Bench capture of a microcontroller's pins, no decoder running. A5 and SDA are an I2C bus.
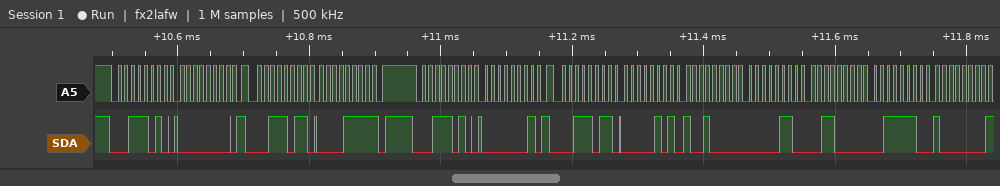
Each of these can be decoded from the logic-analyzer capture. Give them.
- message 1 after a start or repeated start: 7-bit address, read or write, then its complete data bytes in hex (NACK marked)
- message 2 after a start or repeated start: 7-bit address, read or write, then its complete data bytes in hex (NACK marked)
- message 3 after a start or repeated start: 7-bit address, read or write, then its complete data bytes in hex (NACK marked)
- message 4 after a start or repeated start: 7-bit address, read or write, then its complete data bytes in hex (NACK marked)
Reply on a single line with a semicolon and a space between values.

0x1D write: 00; 0x1D read: 0F NACK; 0x1D write: 01; 0x1D read: 05 90 06 30 3E 80 NACK
